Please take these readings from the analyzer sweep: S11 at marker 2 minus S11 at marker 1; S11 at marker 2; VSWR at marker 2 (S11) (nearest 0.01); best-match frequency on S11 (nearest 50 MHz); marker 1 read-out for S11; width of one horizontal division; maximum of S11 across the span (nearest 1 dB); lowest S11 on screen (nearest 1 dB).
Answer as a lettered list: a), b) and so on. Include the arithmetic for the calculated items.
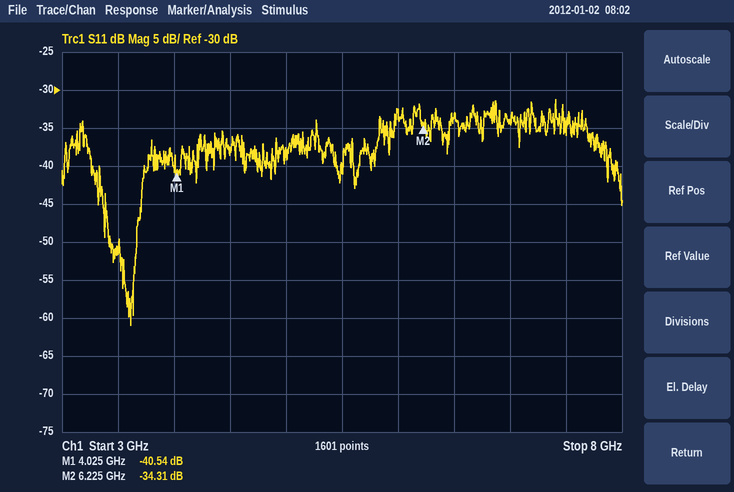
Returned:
a) -34.31 − (-40.54) = 6.23 dB
b) -34.31 dB
c) (1 + 0.0193)/(1 − 0.0193) ≈ 1.04
d) 3.60 GHz
e) -40.54 dB
f) 500 MHz
g) -31 dB
h) -61 dB
